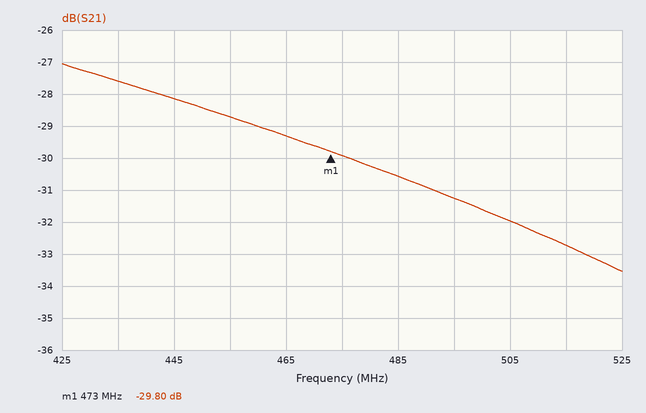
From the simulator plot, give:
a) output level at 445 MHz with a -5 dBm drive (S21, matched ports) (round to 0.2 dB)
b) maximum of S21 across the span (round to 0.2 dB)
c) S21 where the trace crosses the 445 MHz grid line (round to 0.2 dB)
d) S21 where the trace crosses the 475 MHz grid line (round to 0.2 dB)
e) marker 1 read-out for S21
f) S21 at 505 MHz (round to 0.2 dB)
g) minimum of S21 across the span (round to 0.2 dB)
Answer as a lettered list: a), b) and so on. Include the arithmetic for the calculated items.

a) -5 dBm + (-28.2 dB) = -33.2 dBm
b) -27.0 dB
c) -28.2 dB
d) -30.0 dB
e) -29.80 dB
f) -32.0 dB
g) -33.6 dB
